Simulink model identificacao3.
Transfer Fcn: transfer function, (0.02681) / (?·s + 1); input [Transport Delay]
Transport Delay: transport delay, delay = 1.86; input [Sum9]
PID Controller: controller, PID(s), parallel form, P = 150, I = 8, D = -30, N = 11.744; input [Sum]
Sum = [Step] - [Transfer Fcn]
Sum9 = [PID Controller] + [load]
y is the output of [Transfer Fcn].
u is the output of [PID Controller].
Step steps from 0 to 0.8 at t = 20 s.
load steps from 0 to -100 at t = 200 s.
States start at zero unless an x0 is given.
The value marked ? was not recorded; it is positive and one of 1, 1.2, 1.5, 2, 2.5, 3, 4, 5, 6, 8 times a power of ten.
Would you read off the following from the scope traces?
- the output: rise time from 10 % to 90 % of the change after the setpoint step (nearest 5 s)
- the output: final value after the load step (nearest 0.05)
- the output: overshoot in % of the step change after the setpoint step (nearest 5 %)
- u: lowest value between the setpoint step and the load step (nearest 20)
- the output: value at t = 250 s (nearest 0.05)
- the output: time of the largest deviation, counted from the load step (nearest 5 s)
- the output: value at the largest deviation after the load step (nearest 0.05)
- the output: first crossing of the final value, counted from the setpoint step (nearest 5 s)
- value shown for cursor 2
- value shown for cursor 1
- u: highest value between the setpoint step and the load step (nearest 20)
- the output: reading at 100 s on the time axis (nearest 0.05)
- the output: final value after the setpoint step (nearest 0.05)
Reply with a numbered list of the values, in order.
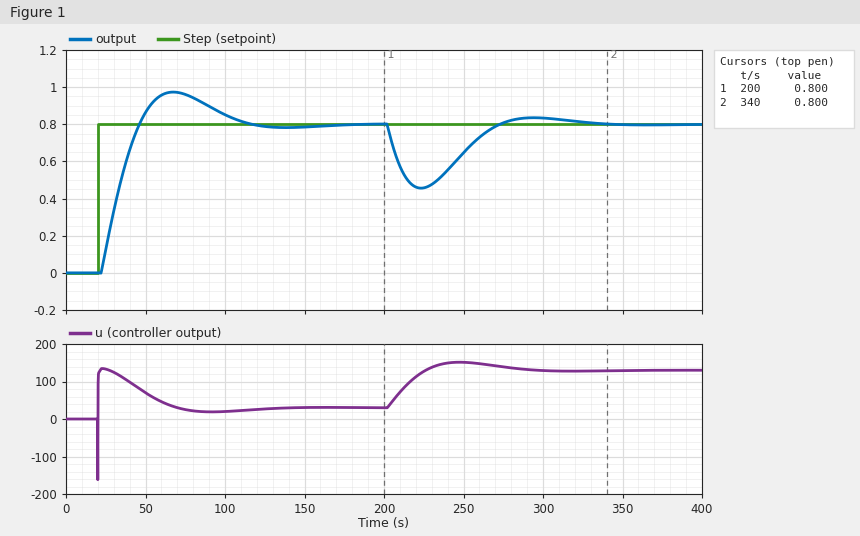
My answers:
1. 20 s
2. 0.80
3. 20 %
4. -160
5. 0.65
6. 25 s
7. 0.45
8. 25 s
9. 0.800
10. 0.800
11. 140
12. 0.85
13. 0.80
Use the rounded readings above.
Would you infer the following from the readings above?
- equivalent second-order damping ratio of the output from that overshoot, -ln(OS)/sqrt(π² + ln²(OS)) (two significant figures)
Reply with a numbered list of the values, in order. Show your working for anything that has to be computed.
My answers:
1. ln(0.2) = -1.609; 1.609 / sqrt(9.870 + 2.590) = 0.46
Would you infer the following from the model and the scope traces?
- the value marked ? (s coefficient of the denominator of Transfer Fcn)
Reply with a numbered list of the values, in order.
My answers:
1. 80
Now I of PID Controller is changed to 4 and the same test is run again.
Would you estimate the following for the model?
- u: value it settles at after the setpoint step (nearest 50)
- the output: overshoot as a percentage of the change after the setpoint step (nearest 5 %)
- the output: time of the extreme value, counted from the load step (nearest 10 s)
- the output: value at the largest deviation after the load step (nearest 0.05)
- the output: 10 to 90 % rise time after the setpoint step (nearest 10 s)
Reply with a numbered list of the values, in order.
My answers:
1. 50
2. 10 %
3. 30 s
4. 0.40
5. 30 s
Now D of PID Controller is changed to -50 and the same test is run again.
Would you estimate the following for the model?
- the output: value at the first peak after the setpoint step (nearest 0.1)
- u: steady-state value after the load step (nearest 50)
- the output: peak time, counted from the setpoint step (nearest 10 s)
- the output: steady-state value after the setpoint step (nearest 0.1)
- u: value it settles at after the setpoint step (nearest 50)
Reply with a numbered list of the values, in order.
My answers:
1. 1.0
2. 150
3. 50 s
4. 0.8
5. 50
